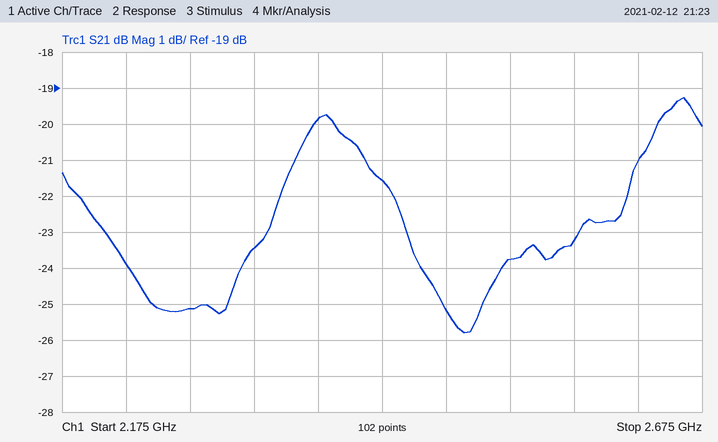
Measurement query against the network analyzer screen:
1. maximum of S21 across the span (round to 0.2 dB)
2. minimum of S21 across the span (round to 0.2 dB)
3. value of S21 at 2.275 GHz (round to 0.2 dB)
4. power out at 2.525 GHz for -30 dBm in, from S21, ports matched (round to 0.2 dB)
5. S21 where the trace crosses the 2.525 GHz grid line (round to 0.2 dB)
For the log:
-19.2 dB
-25.8 dB
-25.2 dB
-53.8 dBm
-23.8 dB
